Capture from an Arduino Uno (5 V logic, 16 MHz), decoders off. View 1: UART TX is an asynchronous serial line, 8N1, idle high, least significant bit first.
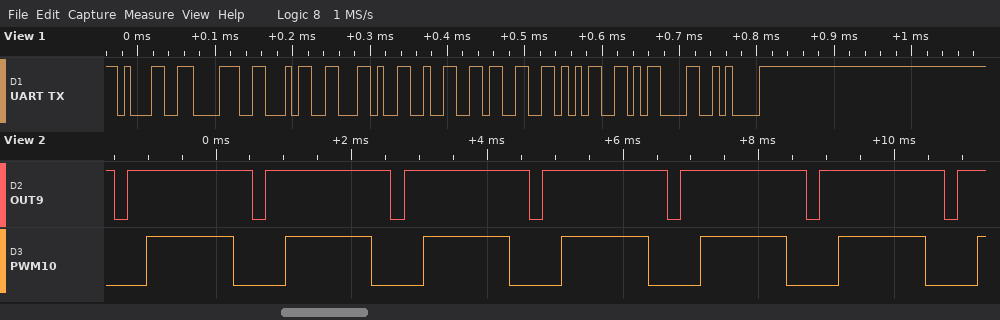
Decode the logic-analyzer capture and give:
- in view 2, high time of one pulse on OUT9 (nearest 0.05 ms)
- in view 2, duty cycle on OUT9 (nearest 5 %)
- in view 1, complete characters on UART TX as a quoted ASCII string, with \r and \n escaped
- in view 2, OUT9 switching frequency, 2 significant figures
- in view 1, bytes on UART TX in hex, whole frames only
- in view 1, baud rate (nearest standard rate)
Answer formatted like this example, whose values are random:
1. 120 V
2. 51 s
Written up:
1. 1.85 ms
2. 90 %
3. "184,235\r\n"
4. 490 Hz
5. 31 38 34 2C 32 33 35 0D 0A
6. 115200 baud
